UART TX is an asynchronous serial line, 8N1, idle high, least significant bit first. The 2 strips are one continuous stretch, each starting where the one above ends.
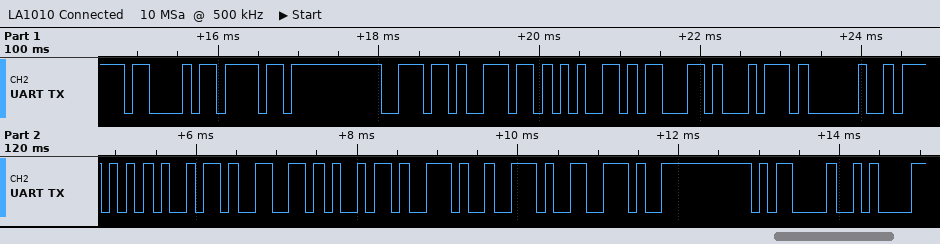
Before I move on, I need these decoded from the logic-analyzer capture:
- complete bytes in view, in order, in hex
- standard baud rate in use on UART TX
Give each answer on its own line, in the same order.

0x43 0x6F 0x6E 0x6E 0x65 0x63 0x74 0x20 0x57 0x69 0x66 0x69 0x2E 0x2E 0x2E 0x0D 0x0A
9600 baud
